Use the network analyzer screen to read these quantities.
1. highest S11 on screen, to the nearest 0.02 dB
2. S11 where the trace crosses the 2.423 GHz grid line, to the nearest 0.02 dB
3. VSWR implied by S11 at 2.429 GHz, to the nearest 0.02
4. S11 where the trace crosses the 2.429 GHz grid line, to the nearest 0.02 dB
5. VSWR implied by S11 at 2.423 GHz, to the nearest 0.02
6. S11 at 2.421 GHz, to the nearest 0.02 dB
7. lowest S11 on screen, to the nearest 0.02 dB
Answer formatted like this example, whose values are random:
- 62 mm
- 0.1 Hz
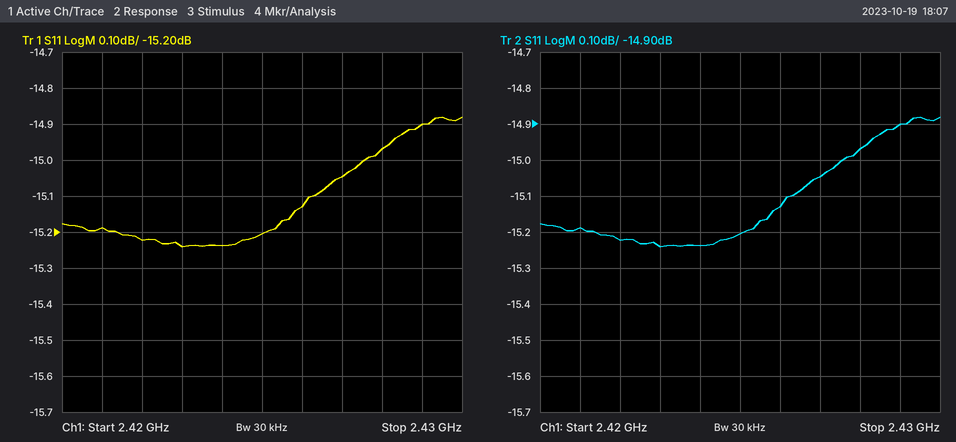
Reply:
- -14.88 dB
- -15.24 dB
- 1.44
- -14.90 dB
- 1.42
- -15.18 dB
- -15.24 dB
